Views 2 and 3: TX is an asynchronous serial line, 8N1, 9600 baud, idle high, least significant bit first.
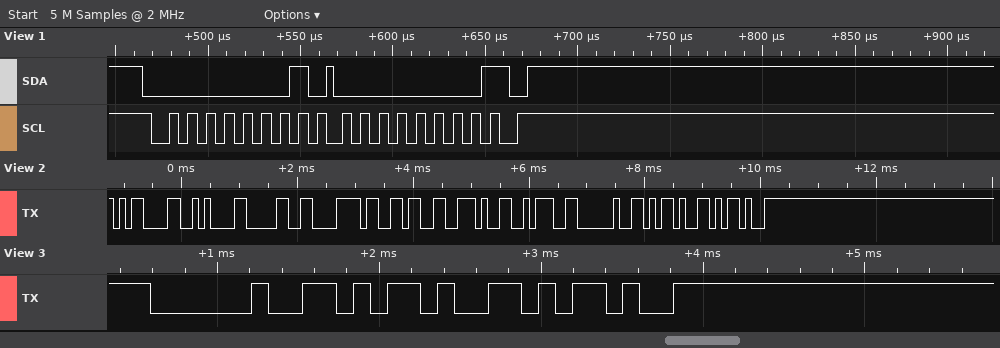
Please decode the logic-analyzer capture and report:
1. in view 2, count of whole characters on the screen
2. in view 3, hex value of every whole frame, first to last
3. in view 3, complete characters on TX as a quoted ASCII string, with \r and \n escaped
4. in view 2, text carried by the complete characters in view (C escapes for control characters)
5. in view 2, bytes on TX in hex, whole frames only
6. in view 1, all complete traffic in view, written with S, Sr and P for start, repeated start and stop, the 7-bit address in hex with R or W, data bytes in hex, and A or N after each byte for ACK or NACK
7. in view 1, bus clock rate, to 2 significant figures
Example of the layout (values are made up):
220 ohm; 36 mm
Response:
10; 20 2D 2D; " --"; "\r\n0x6.: --"; 0D 0A 30 78 36 2E 3A 20 2D 2D; S 00R A 00 N P; 100 kHz
